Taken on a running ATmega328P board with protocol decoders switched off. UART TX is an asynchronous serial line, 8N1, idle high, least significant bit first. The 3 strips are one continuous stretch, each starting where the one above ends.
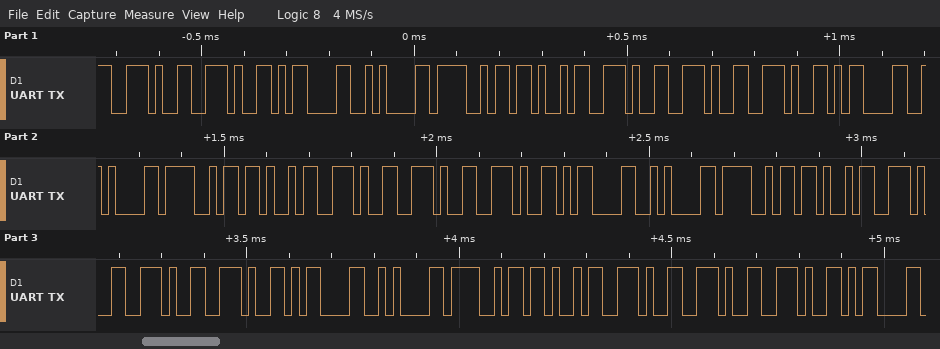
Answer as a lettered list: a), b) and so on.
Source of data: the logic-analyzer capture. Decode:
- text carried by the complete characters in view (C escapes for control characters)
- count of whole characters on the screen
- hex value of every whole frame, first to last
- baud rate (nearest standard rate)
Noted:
a) "..\r\nOK...\r\nOK...\r\nOK...\r\nOK...\r"
b) 31
c) 0x2E 0x2E 0x0D 0x0A 0x4F 0x4B 0x2E 0x2E 0x2E 0x0D 0x0A 0x4F 0x4B 0x2E 0x2E 0x2E 0x0D 0x0A 0x4F 0x4B 0x2E 0x2E 0x2E 0x0D 0x0A 0x4F 0x4B 0x2E 0x2E 0x2E 0x0D
d) 57600 baud
